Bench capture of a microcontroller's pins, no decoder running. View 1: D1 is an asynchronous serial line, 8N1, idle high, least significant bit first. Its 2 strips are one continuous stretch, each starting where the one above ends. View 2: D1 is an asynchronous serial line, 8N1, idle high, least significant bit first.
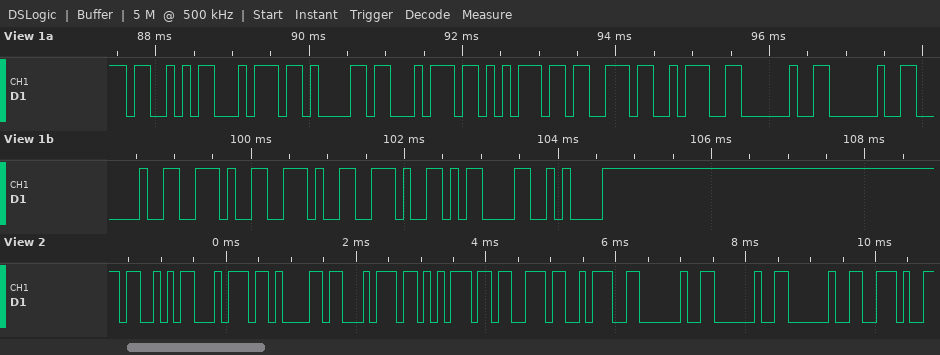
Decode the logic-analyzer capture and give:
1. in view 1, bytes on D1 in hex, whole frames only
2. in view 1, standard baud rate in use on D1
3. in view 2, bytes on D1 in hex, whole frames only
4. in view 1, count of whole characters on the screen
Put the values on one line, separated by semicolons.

0x53 0x74 0x61 0x74 0x75 0x73 0x3A 0x20 0x20 0x20 0x2E 0x2E 0x2E 0x0D 0x0A; 9600 baud; 0x53 0x74 0x61 0x74 0x75 0x73 0x3A 0x20 0x20 0x20 0x2E; 15
